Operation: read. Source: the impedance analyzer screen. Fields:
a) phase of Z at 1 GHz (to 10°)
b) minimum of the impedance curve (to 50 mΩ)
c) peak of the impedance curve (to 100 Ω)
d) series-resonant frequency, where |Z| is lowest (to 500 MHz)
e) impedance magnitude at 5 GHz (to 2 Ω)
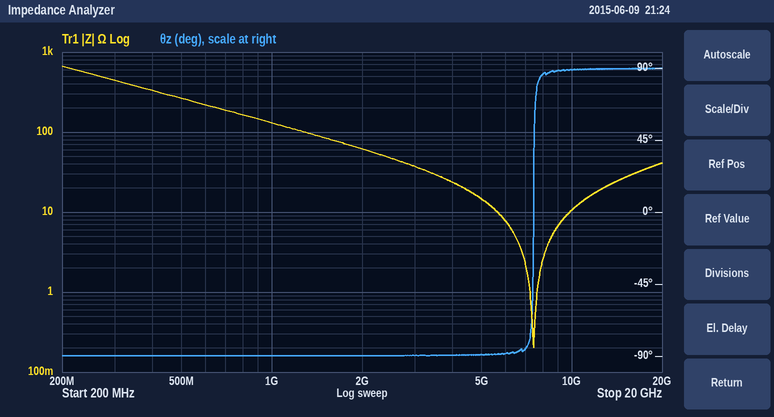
-90°
200 mΩ
700 Ω
7.5 GHz
14 Ω
